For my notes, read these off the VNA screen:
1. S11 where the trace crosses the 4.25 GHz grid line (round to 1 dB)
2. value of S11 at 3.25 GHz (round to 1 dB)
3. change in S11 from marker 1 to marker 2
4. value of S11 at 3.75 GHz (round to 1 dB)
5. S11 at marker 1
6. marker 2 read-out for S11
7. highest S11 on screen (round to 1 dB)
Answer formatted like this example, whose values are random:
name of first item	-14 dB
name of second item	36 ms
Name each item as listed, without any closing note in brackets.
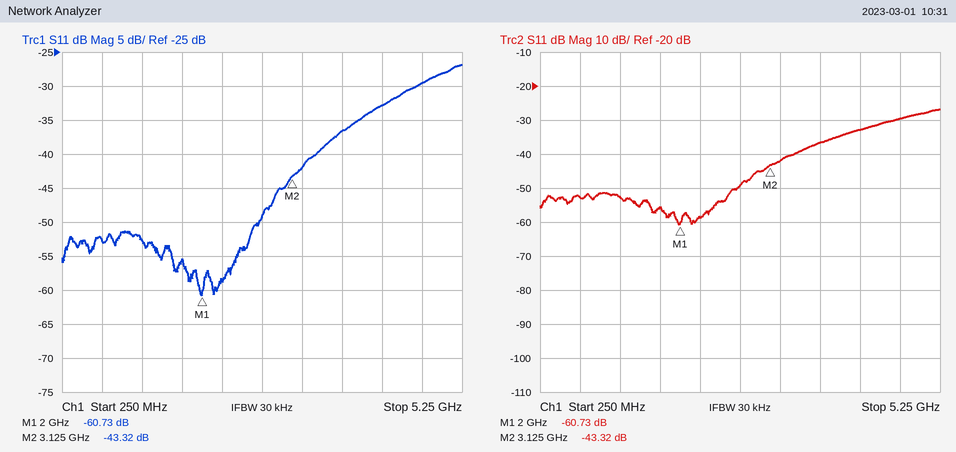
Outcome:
S11 where the trace crosses the 4.25 GHz grid line	-33 dB
value of S11 at 3.25 GHz	-42 dB
change in S11 from marker 1 to marker 2	17.41 dB
value of S11 at 3.75 GHz	-37 dB
S11 at marker 1	-60.73 dB
marker 2 read-out for S11	-43.32 dB
highest S11 on screen	-27 dB
